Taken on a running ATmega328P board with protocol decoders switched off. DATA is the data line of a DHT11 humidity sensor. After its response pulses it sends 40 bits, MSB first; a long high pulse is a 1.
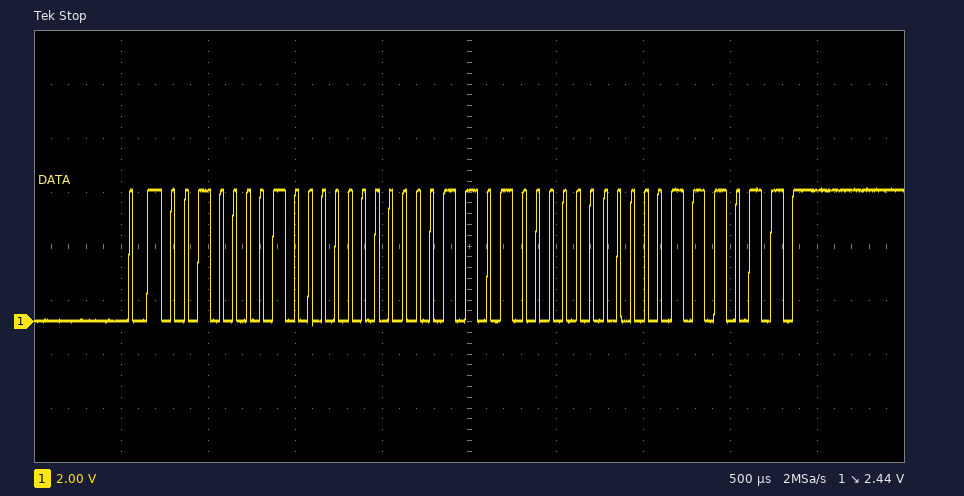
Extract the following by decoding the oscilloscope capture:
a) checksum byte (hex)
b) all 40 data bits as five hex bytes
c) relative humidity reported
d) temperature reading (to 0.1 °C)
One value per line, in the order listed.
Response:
0x3B
21 00 1A 00 3B
33 %
26.0 °C
